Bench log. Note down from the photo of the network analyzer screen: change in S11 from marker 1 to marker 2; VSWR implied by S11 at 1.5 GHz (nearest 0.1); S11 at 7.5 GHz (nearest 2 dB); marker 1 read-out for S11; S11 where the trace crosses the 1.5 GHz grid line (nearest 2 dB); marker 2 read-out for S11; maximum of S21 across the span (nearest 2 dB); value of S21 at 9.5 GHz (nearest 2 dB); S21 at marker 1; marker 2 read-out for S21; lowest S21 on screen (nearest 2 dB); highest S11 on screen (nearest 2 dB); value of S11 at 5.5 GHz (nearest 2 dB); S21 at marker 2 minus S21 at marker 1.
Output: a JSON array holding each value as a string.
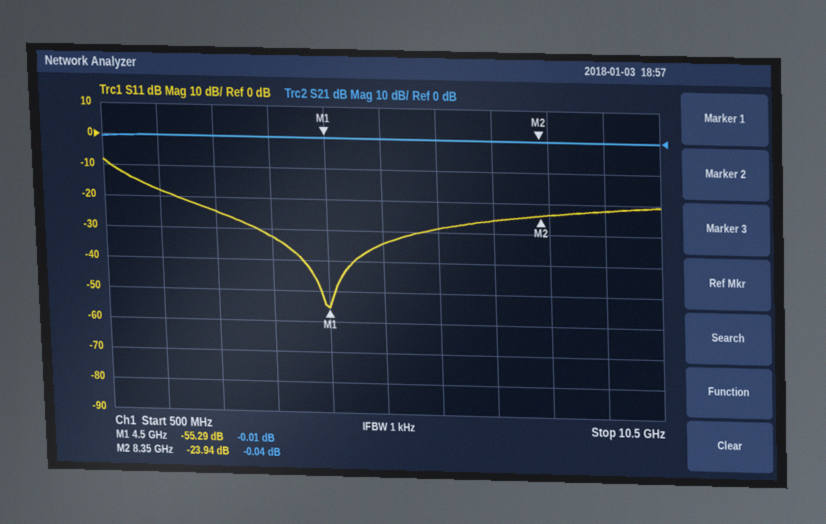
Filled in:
["31.35 dB", "1.3", "-26 dB", "-55.29 dB", "-18 dB", "-23.94 dB", "0 dB", "0 dB", "-0.01 dB", "-0.04 dB", "0 dB", "-8 dB", "-34 dB", "-0.03 dB"]
